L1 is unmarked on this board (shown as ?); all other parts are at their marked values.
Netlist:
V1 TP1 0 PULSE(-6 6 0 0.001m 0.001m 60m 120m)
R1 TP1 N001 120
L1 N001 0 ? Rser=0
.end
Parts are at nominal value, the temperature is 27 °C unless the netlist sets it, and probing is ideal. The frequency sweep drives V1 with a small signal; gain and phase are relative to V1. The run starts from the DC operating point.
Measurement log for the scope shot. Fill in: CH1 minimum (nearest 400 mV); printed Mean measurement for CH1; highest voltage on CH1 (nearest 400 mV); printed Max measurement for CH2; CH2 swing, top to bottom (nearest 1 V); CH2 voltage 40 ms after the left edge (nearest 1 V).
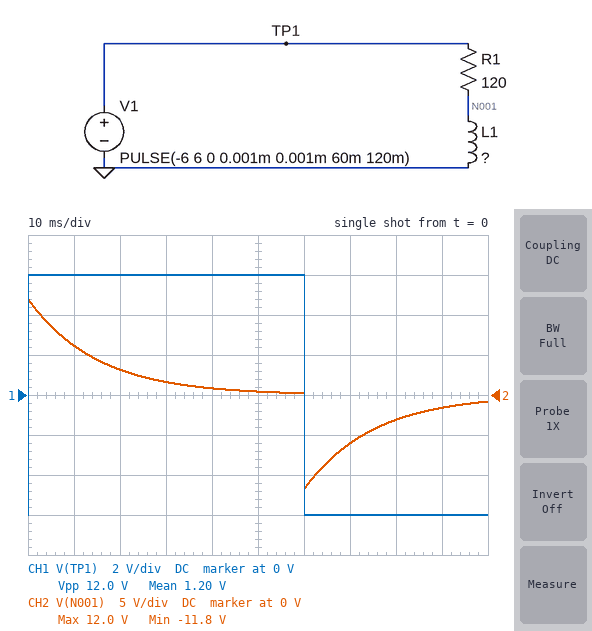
-6.0 V
1.20 V
6.0 V
12.0 V
24 V
1 V
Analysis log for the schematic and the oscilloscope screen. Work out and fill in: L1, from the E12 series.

1.8 H
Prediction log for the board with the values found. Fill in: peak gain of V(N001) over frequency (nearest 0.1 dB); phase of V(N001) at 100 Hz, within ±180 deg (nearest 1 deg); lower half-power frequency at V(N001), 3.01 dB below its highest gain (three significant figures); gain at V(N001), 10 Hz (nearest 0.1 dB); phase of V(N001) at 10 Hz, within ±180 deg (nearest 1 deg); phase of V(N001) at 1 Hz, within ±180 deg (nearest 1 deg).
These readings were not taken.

0 dB
6 deg
10.6 Hz
-3.3 dB
47 deg
85 deg
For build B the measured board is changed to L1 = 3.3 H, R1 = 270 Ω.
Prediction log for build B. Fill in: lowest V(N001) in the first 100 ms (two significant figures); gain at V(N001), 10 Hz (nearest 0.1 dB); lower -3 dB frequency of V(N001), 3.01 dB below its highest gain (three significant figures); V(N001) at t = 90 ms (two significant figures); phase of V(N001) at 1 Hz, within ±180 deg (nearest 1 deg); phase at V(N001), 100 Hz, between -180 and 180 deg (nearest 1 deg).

-12 V
-4.3 dB
13.0 Hz
-1.0 V
86 deg
7 deg
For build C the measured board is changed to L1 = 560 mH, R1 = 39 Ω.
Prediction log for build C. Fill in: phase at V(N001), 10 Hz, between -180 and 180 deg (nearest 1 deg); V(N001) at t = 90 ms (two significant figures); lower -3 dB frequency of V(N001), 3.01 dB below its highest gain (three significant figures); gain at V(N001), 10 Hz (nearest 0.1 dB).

48 deg
-1.5 V
11.1 Hz
-3.5 dB
